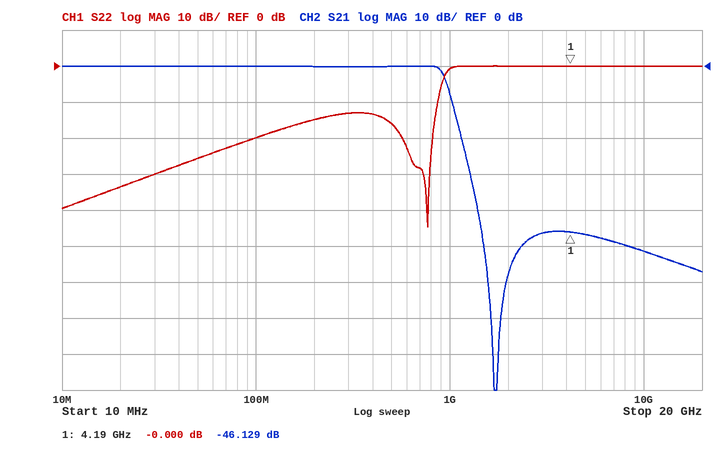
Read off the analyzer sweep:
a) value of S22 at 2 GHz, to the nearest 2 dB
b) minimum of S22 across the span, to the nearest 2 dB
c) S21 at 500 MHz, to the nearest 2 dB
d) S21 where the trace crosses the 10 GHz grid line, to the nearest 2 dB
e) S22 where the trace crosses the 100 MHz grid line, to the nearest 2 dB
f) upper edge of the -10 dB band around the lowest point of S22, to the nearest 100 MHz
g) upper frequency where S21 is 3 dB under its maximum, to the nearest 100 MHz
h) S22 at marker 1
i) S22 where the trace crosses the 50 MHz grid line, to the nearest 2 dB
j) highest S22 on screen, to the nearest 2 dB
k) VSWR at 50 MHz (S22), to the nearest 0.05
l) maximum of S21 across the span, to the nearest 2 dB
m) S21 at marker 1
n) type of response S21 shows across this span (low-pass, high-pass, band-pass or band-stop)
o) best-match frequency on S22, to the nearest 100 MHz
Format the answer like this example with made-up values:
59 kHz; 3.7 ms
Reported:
0 dB; -44 dB; 0 dB; -52 dB; -20 dB; 900 MHz; 900 MHz; -0.000 dB; -26 dB; 0 dB; 1.10; 0 dB; -46.129 dB; low-pass; 800 MHz
